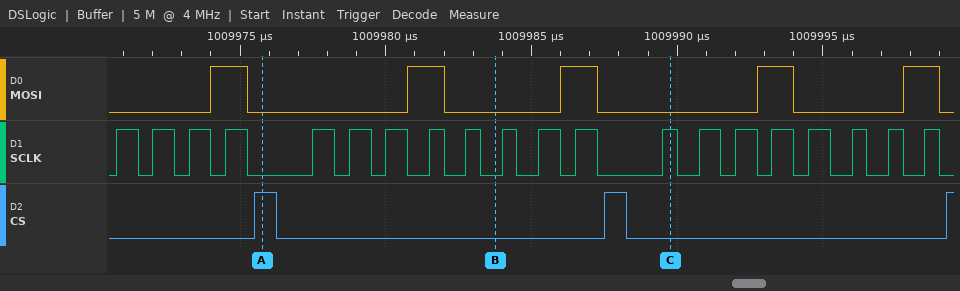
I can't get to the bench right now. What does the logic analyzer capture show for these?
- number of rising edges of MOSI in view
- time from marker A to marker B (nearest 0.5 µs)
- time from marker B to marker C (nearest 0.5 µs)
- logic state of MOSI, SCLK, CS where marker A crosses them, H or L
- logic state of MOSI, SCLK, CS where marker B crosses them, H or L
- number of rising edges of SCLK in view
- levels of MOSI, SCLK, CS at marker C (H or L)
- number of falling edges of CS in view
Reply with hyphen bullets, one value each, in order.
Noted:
- 5
- 8 µs
- 6 µs
- MOSI=L, SCLK=L, CS=H
- MOSI=L, SCLK=L, CS=L
- 20
- MOSI=L, SCLK=H, CS=L
- 2
